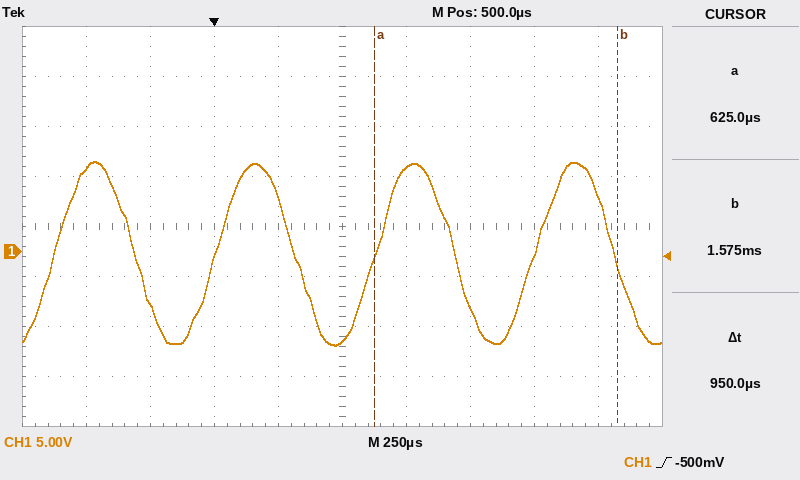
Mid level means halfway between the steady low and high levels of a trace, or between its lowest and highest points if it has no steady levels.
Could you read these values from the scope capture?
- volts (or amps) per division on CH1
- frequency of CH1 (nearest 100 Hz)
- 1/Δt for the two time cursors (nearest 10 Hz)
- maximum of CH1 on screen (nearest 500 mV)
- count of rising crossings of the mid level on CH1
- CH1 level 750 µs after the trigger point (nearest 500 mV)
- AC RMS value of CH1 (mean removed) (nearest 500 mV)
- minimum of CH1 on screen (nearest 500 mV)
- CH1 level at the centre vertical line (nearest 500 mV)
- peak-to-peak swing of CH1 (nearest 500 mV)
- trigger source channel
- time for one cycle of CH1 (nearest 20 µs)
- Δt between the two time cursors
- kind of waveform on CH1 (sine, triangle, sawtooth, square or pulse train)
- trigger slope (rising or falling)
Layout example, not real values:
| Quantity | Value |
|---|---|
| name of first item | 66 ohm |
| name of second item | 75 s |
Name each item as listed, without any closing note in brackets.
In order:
| Quantity | Value |
|---|---|
| volts (or amps) per division on CH1 | 5 V |
| frequency of CH1 | 1.6 kHz |
| 1/Δt for the two time cursors | 1.05 kHz |
| maximum of CH1 on screen | 9.0 V |
| count of rising crossings of the mid level on CH1 | 4 |
| CH1 level 750 µs after the trigger point | 8.5 V |
| AC RMS value of CH1 (mean removed) | 6.5 V |
| minimum of CH1 on screen | -9.5 V |
| CH1 level at the centre vertical line | -9.0 V |
| peak-to-peak swing of CH1 | 18.5 V |
| trigger source channel | CH1 |
| time for one cycle of CH1 | 620 µs |
| Δt between the two time cursors | 950 µs |
| kind of waveform on CH1 | sine |
| trigger slope | rising |
